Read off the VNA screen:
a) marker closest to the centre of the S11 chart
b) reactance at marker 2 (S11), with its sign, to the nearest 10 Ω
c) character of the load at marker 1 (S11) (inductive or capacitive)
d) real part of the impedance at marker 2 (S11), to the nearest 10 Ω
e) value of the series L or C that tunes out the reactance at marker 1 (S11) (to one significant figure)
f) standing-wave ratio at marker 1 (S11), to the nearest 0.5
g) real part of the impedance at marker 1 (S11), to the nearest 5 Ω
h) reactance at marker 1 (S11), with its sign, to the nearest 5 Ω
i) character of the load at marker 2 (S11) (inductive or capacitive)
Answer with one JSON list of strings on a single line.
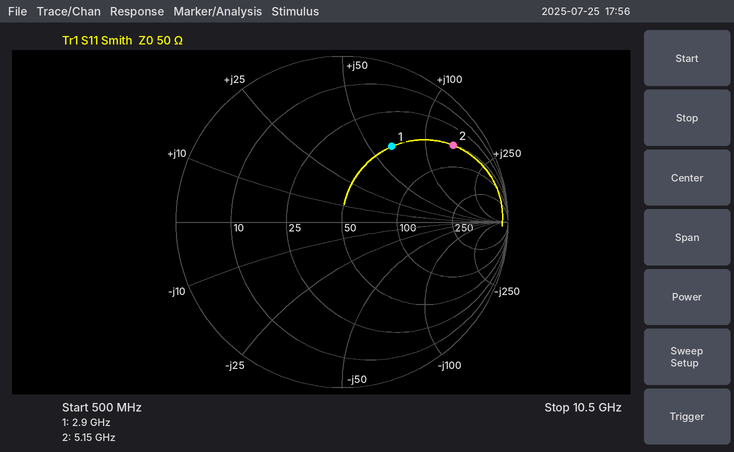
["marker 1", "+140 Ω", "inductive", "50 Ω", "800 fF", "3.5", "50 Ω", "+65 Ω", "inductive"]
